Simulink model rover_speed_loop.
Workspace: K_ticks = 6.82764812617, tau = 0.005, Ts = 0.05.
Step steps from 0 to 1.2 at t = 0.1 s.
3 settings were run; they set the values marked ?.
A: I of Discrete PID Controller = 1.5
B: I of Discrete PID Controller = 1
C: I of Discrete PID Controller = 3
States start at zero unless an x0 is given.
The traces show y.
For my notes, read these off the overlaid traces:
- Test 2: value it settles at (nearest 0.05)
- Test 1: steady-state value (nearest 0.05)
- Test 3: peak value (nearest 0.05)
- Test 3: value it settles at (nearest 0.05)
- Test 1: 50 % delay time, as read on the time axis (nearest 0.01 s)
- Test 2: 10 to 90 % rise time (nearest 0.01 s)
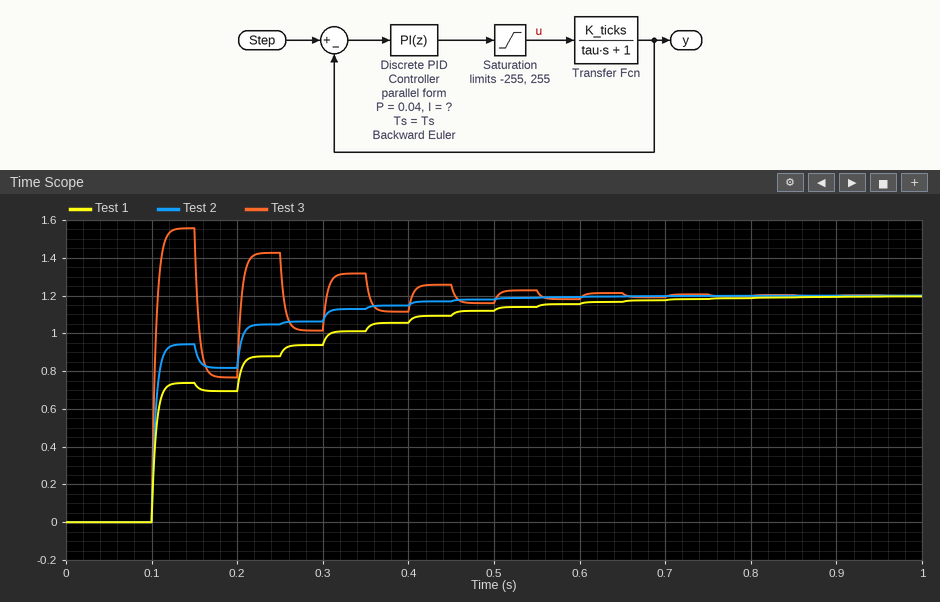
1.20
1.20
1.55
1.20
0.11 s
0.20 s
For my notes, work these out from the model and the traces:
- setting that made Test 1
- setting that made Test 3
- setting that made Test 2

B
C
A
